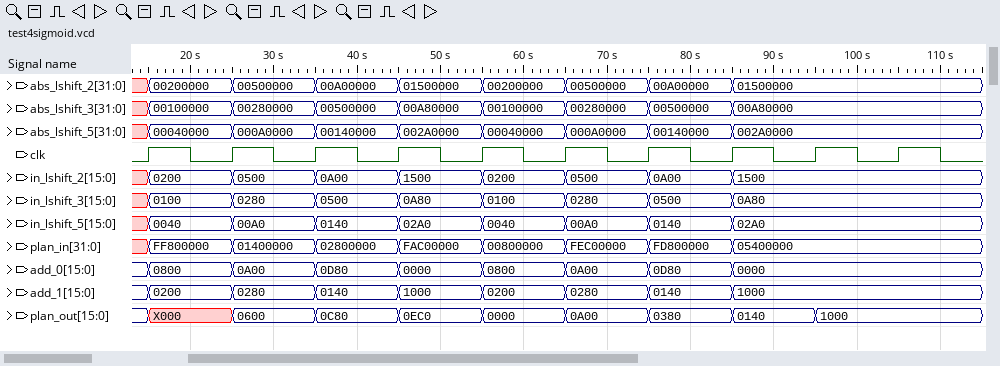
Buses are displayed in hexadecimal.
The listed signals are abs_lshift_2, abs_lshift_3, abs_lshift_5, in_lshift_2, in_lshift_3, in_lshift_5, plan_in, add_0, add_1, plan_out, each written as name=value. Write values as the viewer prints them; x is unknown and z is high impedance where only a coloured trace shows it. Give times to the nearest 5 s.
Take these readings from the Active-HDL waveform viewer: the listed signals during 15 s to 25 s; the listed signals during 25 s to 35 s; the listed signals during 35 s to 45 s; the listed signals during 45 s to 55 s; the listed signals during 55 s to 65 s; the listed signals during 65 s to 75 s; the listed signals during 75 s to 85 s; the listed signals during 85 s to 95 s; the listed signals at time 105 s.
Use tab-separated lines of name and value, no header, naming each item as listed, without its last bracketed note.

the listed signals during 15 s to 25 s	abs_lshift_2=00200000, abs_lshift_3=00100000, abs_lshift_5=00040000, in_lshift_2=0200, in_lshift_3=0100, in_lshift_5=0040, plan_in=FF800000, add_0=0800, add_1=0200, plan_out=X000
the listed signals during 25 s to 35 s	abs_lshift_2=00500000, abs_lshift_3=00280000, abs_lshift_5=000A0000, in_lshift_2=0500, in_lshift_3=0280, in_lshift_5=00A0, plan_in=01400000, add_0=0A00, add_1=0280, plan_out=0600
the listed signals during 35 s to 45 s	abs_lshift_2=00A00000, abs_lshift_3=00500000, abs_lshift_5=00140000, in_lshift_2=0A00, in_lshift_3=0500, in_lshift_5=0140, plan_in=02800000, add_0=0D80, add_1=0140, plan_out=0C80
the listed signals during 45 s to 55 s	abs_lshift_2=01500000, abs_lshift_3=00A80000, abs_lshift_5=002A0000, in_lshift_2=1500, in_lshift_3=0A80, in_lshift_5=02A0, plan_in=FAC00000, add_0=0000, add_1=1000, plan_out=0EC0
the listed signals during 55 s to 65 s	abs_lshift_2=00200000, abs_lshift_3=00100000, abs_lshift_5=00040000, in_lshift_2=0200, in_lshift_3=0100, in_lshift_5=0040, plan_in=00800000, add_0=0800, add_1=0200, plan_out=0000
the listed signals during 65 s to 75 s	abs_lshift_2=00500000, abs_lshift_3=00280000, abs_lshift_5=000A0000, in_lshift_2=0500, in_lshift_3=0280, in_lshift_5=00A0, plan_in=FEC00000, add_0=0A00, add_1=0280, plan_out=0A00
the listed signals during 75 s to 85 s	abs_lshift_2=00A00000, abs_lshift_3=00500000, abs_lshift_5=00140000, in_lshift_2=0A00, in_lshift_3=0500, in_lshift_5=0140, plan_in=FD800000, add_0=0D80, add_1=0140, plan_out=0380
the listed signals during 85 s to 95 s	abs_lshift_2=01500000, abs_lshift_3=00A80000, abs_lshift_5=002A0000, in_lshift_2=1500, in_lshift_3=0A80, in_lshift_5=02A0, plan_in=05400000, add_0=0000, add_1=1000, plan_out=0140
the listed signals at time 105 s	abs_lshift_2=01500000, abs_lshift_3=00A80000, abs_lshift_5=002A0000, in_lshift_2=1500, in_lshift_3=0A80, in_lshift_5=02A0, plan_in=05400000, add_0=0000, add_1=1000, plan_out=1000
